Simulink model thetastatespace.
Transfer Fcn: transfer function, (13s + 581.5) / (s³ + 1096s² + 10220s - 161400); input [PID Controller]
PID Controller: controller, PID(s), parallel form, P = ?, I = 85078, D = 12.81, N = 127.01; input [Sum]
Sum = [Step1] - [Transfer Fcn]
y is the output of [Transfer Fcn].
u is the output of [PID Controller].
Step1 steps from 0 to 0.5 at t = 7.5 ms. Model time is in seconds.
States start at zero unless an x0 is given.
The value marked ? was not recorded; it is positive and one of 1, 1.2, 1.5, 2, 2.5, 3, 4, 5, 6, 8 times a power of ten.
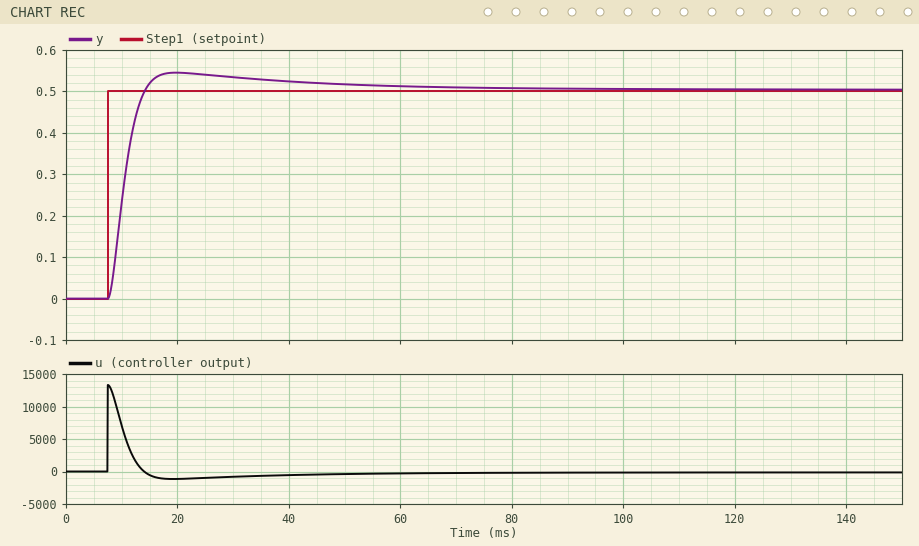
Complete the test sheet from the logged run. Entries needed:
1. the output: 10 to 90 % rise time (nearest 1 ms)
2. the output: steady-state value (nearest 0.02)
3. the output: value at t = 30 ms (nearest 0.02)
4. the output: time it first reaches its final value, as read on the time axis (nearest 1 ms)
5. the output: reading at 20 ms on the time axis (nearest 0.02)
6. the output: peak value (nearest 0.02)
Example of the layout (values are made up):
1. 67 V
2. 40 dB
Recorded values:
1. 4 ms
2. 0.50
3. 0.54
4. 14 ms
5. 0.54
6. 0.54
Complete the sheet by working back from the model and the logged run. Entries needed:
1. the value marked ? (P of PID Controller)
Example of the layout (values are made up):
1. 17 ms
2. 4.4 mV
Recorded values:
1. 25000
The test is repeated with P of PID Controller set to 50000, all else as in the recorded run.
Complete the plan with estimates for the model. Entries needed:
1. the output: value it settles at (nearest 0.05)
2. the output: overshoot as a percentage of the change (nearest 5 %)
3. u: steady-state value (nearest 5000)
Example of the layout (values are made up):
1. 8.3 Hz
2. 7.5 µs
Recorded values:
1. 0.50
2. 10 %
3. 0
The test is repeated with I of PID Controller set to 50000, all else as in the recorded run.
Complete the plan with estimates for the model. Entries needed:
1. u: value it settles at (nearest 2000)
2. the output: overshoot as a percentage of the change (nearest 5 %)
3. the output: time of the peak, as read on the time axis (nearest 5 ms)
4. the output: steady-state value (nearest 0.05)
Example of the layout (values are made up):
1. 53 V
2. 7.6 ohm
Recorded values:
1. 0
2. 10 %
3. 20 ms
4. 0.50
